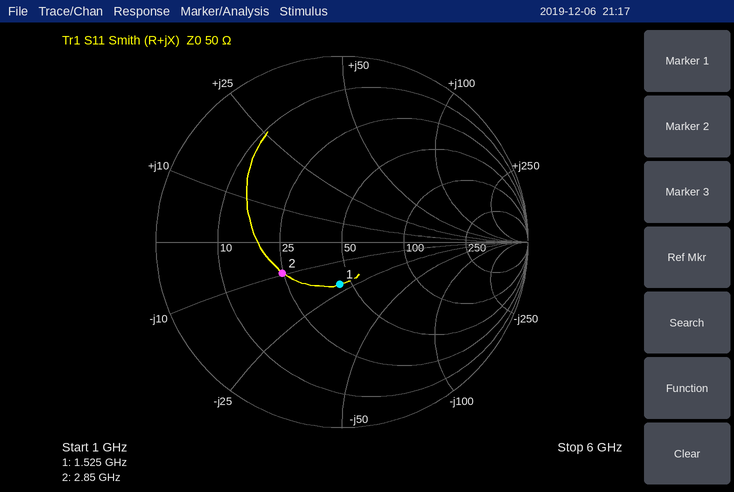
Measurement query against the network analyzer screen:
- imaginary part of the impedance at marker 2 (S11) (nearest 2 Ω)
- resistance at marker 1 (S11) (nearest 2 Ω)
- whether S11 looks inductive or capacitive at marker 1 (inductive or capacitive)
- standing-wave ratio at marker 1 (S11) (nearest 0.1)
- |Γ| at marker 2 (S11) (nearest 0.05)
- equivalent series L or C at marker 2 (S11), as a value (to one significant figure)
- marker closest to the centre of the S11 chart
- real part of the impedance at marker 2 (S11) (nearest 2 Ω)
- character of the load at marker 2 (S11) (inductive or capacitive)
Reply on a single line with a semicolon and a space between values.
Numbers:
-10 Ω; 44 Ω; capacitive; 1.6; 0.35; 6 pF; marker 1; 24 Ω; capacitive
